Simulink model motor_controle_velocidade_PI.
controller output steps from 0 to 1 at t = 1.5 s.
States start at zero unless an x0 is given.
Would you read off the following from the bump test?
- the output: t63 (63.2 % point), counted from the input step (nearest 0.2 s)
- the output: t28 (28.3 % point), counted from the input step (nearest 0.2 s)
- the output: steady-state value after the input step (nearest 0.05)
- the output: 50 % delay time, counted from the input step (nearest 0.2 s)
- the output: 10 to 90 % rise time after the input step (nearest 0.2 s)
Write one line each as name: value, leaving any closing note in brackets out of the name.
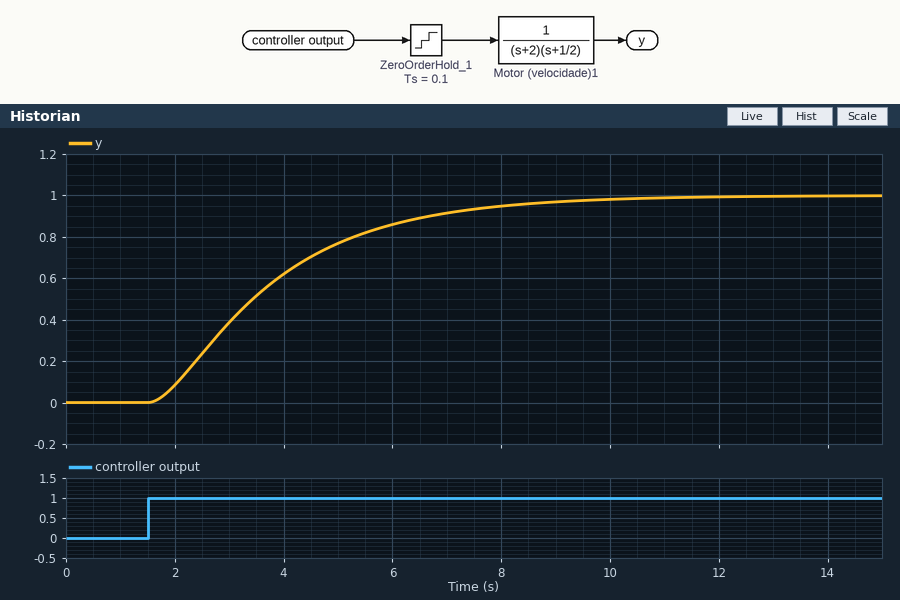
the output: t63 (63.2 % point), counted from the input step: 2.6 s
the output: t28 (28.3 % point), counted from the input step: 1.2 s
the output: steady-state value after the input step: 1.00
the output: 50 % delay time, counted from the input step: 2.0 s
the output: 10 to 90 % rise time after the input step: 4.6 s
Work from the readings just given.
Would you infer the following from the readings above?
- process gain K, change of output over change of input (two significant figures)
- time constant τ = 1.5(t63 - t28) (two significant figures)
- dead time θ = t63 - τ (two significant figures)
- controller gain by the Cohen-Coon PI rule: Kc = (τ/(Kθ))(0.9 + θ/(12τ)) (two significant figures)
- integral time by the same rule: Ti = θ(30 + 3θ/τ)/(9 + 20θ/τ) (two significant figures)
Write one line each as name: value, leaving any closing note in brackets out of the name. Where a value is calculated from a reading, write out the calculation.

process gain K, change of output over change of input: (1 - 0) / 1 = 1.0
time constant τ = 1.5(t63 - t28): 1.5 × (2.6 - 1.2) = 2.1 s
dead time θ = t63 - τ: 2.6 - 2.1 = 0.50 s
controller gain by the Cohen-Coon PI rule: Kc = (τ/(Kθ))(0.9 + θ/(12τ)): 2.1 / (1 × 0.5) × (0.9 + 0.5 / (12 × 2.1)) = 3.9
integral time by the same rule: Ti = θ(30 + 3θ/τ)/(9 + 20θ/τ): 0.5 × (30 + 3 × 0.5 / 2.1) / (9 + 20 × 0.5 / 2.1) = 1.1 s
